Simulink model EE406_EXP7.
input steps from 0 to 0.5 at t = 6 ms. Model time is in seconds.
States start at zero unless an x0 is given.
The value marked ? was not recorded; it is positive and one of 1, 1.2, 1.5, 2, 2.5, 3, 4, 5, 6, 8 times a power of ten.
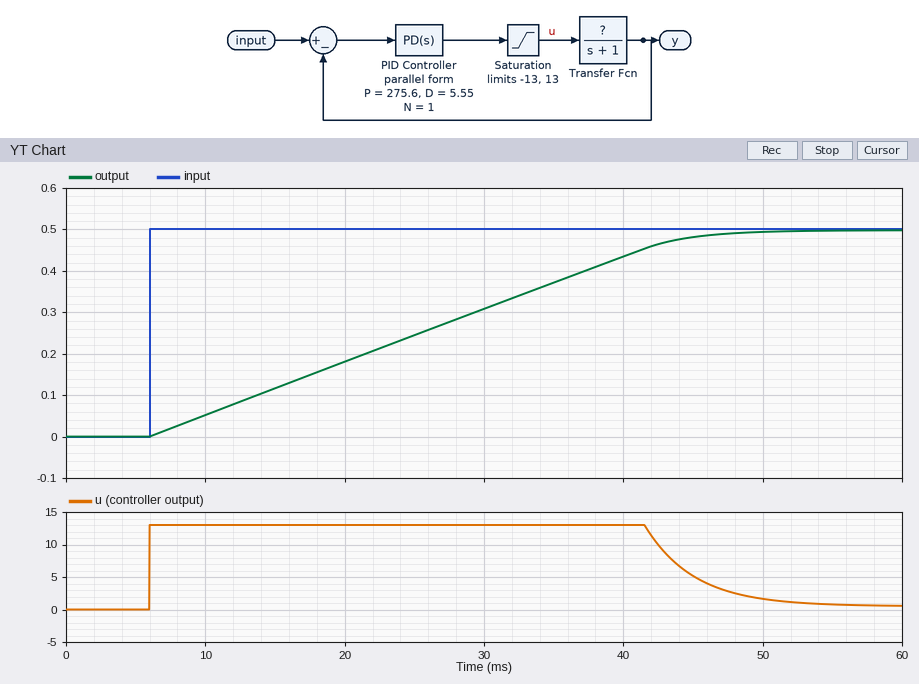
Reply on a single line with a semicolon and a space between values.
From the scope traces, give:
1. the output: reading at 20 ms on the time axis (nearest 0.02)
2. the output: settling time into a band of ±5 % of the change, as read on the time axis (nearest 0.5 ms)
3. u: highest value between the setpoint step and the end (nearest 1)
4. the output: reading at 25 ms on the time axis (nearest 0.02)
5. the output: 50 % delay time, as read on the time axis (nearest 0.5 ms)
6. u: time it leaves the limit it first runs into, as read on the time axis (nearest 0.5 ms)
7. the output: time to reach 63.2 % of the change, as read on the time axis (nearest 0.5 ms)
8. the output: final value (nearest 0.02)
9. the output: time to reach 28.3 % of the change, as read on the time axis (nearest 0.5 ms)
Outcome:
0.18; 43.5 ms; 13; 0.24; 25.5 ms; 41.5 ms; 30.5 ms; 0.50; 17.0 ms
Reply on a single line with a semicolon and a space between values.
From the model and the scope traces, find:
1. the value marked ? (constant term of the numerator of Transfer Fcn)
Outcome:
1
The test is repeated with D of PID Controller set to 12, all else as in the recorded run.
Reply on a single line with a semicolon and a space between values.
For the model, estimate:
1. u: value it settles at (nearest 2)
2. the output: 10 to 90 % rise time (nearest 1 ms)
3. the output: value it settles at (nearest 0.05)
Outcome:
0; 31 ms; 0.50
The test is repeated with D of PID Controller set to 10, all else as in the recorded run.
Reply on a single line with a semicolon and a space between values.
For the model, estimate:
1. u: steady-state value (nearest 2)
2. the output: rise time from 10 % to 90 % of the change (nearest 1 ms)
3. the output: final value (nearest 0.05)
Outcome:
0; 31 ms; 0.50
